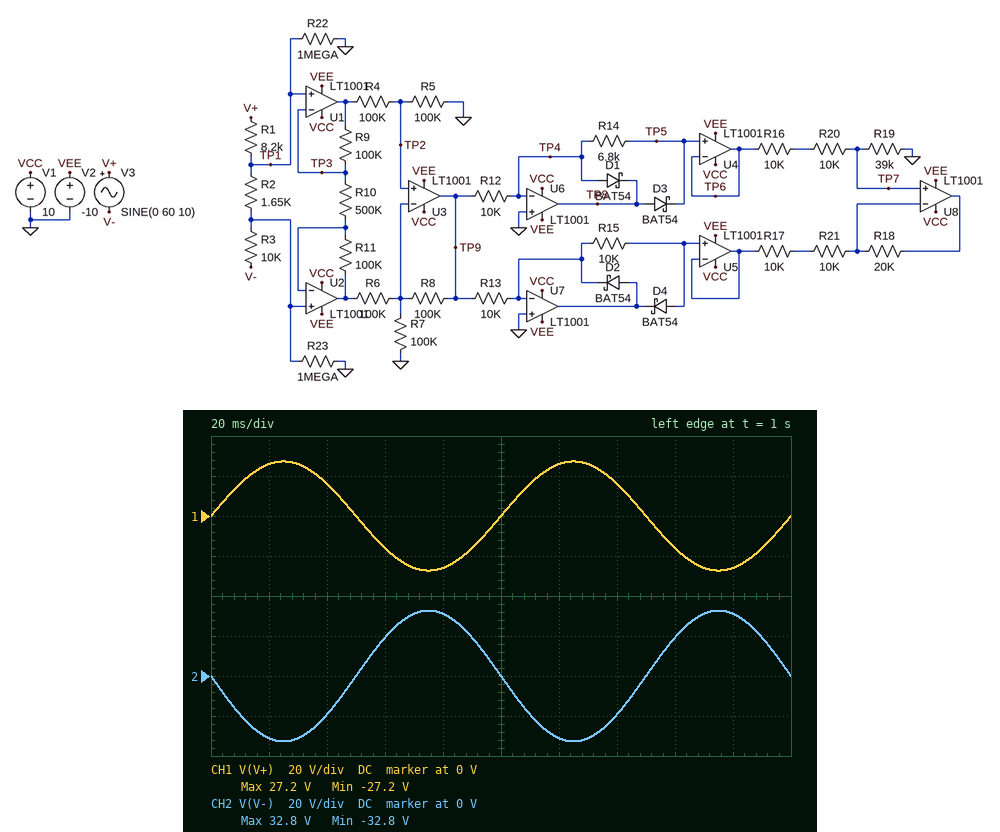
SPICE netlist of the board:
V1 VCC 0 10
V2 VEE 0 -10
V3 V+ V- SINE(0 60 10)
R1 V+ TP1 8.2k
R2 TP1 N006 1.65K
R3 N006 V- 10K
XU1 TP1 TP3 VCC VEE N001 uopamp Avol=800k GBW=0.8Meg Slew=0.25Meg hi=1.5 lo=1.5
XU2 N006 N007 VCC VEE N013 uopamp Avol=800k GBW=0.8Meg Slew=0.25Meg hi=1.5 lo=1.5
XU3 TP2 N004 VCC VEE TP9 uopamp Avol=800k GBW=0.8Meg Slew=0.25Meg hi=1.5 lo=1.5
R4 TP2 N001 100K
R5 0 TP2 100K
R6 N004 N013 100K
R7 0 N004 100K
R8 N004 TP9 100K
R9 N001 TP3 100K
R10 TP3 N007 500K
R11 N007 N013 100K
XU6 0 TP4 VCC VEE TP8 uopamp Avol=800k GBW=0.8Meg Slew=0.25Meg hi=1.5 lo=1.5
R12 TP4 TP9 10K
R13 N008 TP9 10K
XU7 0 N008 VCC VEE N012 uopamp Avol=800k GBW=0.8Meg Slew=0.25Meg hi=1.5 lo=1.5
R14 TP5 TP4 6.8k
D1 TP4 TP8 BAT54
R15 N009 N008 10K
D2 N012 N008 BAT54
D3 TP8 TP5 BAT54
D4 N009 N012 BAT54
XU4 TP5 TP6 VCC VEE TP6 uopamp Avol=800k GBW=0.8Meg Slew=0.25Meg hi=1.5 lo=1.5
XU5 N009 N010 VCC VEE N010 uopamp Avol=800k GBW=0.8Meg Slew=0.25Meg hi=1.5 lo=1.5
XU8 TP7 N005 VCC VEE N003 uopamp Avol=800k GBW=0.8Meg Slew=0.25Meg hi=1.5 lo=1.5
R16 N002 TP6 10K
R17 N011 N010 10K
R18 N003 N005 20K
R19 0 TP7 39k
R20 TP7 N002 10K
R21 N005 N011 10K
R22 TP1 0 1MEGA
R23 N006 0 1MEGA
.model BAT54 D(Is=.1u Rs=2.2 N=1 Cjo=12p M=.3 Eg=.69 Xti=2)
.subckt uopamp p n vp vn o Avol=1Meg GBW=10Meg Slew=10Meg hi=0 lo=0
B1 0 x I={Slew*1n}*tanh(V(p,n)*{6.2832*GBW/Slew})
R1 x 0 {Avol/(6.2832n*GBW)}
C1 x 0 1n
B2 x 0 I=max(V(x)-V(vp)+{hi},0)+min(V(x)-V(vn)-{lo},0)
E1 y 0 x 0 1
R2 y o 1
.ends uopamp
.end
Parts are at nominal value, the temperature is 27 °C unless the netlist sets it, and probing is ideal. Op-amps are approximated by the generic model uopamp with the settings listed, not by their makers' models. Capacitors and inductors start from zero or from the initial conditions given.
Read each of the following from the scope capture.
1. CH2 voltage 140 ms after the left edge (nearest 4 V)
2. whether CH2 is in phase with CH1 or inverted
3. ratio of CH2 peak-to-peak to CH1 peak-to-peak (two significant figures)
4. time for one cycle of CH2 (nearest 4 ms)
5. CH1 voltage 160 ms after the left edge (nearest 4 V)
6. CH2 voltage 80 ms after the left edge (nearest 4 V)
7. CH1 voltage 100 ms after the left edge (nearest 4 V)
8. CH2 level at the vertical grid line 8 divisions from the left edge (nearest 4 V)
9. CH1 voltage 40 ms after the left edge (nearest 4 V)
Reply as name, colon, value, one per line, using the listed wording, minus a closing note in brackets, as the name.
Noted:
CH2 voltage 140 ms after the left edge: -20 V
whether CH2 is in phase with CH1 or inverted: inverted
ratio of CH2 peak-to-peak to CH1 peak-to-peak: 1.2
time for one cycle of CH2: 100 ms
CH1 voltage 160 ms after the left edge: -16 V
CH2 voltage 80 ms after the left edge: 32 V
CH1 voltage 100 ms after the left edge: 0 V
CH2 level at the vertical grid line 8 divisions from the left edge: 20 V
CH1 voltage 40 ms after the left edge: 16 V
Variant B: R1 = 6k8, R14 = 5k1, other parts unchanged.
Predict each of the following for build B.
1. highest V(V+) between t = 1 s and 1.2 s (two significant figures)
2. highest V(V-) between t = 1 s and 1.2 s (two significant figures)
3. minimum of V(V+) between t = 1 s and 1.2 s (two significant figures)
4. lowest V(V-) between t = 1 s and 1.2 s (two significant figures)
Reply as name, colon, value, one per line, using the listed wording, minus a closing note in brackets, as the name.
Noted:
highest V(V+) between t = 1 s and 1.2 s: 25 V
highest V(V-) between t = 1 s and 1.2 s: 35 V
minimum of V(V+) between t = 1 s and 1.2 s: -25 V
lowest V(V-) between t = 1 s and 1.2 s: -35 V
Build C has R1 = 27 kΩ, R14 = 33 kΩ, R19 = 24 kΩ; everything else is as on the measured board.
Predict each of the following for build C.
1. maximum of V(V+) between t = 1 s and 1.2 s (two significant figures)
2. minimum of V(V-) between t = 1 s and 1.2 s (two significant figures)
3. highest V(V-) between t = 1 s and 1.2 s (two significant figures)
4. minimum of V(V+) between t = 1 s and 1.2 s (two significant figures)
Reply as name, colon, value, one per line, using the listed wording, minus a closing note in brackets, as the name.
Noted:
maximum of V(V+) between t = 1 s and 1.2 s: 43 V
minimum of V(V-) between t = 1 s and 1.2 s: -17 V
highest V(V-) between t = 1 s and 1.2 s: 17 V
minimum of V(V+) between t = 1 s and 1.2 s: -43 V
